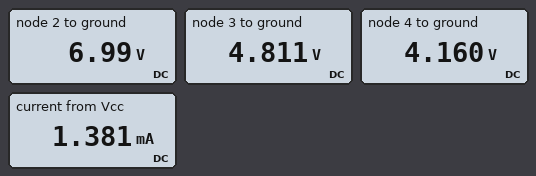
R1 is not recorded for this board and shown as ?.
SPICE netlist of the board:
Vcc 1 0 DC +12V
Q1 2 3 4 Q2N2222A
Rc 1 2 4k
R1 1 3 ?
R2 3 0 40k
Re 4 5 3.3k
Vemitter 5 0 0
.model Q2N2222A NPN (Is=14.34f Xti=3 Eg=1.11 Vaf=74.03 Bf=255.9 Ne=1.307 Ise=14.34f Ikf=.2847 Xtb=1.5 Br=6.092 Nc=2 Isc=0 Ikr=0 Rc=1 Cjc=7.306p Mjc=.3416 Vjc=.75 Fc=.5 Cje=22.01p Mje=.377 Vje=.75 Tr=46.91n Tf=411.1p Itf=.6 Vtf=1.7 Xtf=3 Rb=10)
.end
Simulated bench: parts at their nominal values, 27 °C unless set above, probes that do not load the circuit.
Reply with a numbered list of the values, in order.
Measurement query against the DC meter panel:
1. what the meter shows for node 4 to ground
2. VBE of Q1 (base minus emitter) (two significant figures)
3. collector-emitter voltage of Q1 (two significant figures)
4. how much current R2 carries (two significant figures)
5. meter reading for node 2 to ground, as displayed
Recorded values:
1. 4.160 V
2. 650 mV
3. 2.8 V
4. 120 µA
5. 6.99 V
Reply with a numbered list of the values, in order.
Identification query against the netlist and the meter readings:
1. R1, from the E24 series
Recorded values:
1. 56 kΩ
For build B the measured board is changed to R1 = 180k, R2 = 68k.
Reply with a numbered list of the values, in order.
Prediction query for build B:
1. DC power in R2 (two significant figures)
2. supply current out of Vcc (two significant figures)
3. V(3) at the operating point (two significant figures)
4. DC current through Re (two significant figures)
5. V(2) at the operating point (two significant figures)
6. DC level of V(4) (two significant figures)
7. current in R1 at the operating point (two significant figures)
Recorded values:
1. 140 µW
2. 780 µA
3. 3.1 V
4. 730 µA
5. 9.1 V
6. 2.4 V
7. 50 µA
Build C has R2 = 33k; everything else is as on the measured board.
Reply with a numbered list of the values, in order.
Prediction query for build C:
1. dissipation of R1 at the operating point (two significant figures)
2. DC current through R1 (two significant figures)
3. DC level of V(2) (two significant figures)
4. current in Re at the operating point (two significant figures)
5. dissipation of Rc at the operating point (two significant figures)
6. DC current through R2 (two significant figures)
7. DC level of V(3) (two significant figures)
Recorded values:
1. 1.1 mW
2. 140 µA
3. 7.6 V
4. 1.1 mA
5. 4.8 mW
6. 130 µA
7. 4.3 V
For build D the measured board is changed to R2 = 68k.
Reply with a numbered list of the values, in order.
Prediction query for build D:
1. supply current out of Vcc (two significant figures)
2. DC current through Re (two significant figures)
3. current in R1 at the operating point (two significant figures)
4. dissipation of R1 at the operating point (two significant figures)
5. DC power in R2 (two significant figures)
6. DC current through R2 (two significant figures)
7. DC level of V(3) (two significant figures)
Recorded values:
1. 1.7 mA
2. 1.6 mA
3. 110 µA
4. 630 µW
5. 540 µW
6. 89 µA
7. 6.1 V
